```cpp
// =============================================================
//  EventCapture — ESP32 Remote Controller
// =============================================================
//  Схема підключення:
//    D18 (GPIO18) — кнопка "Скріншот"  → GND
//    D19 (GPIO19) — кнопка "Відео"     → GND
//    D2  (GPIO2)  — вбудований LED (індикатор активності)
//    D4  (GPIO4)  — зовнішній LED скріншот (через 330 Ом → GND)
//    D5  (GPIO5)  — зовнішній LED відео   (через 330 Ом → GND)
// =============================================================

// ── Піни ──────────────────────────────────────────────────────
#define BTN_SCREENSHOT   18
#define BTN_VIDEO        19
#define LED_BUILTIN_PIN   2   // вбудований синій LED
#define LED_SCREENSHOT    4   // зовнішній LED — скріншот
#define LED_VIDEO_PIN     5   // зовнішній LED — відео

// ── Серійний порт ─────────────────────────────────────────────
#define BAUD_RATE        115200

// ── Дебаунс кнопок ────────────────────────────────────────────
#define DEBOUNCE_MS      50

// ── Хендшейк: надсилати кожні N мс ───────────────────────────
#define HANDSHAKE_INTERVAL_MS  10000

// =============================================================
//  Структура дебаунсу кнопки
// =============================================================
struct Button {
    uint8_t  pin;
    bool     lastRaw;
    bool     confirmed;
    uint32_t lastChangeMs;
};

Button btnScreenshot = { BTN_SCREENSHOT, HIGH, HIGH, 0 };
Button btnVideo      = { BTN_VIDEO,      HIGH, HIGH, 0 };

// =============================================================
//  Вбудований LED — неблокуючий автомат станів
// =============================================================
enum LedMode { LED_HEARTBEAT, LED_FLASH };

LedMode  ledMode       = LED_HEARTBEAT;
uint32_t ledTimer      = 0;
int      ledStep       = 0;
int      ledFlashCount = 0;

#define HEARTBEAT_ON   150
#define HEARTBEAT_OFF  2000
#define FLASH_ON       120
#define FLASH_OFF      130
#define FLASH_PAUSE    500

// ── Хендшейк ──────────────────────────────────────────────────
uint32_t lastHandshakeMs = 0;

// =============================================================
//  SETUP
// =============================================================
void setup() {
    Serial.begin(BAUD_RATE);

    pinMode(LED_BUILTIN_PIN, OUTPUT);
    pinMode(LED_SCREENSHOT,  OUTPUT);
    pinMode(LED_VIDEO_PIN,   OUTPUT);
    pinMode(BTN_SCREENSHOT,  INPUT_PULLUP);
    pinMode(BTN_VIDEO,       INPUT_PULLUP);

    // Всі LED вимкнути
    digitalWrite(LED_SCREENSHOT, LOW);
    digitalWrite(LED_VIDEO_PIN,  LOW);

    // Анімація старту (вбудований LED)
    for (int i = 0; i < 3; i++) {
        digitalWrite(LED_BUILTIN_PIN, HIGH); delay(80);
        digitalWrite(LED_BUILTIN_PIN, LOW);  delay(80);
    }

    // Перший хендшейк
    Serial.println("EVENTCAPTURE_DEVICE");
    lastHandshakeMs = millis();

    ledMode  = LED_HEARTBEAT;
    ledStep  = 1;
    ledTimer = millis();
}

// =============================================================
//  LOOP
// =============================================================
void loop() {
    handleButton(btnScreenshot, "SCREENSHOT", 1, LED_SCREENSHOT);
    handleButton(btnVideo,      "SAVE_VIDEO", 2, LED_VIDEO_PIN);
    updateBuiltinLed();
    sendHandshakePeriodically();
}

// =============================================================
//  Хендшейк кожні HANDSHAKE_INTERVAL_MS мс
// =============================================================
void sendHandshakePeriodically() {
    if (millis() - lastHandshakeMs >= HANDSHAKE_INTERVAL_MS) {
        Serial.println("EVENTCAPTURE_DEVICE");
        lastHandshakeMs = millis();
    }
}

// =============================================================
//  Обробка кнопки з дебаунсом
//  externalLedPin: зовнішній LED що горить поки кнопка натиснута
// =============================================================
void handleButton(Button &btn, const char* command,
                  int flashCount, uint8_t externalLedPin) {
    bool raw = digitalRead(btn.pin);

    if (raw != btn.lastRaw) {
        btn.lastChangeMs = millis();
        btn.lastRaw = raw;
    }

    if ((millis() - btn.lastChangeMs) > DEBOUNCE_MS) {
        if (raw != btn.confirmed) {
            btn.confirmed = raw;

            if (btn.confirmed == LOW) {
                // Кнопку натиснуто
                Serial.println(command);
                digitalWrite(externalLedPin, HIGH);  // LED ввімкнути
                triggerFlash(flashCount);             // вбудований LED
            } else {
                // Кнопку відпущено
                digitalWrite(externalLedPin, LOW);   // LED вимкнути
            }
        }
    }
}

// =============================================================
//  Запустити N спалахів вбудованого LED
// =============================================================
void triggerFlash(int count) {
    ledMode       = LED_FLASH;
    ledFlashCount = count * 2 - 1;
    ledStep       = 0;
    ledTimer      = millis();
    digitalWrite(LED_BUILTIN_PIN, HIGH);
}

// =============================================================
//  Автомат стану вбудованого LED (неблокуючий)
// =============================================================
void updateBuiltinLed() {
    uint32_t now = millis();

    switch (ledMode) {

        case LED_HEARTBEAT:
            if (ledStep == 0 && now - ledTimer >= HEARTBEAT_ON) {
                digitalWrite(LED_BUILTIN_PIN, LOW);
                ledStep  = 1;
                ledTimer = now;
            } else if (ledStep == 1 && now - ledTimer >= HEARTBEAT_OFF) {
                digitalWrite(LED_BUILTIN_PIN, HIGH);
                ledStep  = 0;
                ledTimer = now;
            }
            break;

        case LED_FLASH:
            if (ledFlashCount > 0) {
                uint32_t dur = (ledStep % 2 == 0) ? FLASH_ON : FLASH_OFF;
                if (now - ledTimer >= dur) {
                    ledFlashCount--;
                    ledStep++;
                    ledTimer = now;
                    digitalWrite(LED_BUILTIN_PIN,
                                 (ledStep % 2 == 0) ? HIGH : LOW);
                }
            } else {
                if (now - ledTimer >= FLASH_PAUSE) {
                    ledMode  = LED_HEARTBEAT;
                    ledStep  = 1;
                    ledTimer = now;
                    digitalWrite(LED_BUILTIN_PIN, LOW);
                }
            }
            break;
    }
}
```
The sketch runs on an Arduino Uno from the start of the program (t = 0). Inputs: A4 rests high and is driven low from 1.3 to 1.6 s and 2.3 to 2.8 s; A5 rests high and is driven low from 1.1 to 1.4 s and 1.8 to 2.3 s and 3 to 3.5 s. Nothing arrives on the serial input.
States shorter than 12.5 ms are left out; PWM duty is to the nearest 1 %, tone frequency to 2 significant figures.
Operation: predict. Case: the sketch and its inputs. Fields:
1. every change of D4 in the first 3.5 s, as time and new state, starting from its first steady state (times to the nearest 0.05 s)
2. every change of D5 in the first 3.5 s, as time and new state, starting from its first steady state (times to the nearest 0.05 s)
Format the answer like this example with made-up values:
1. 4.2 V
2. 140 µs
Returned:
1. 0 s low; 1.35 s high; 1.65 s low; 2.35 s high; 2.85 s low
2. 0 s low; 1.15 s high; 1.45 s low; 1.85 s high; 2.35 s low; 3.05 s high
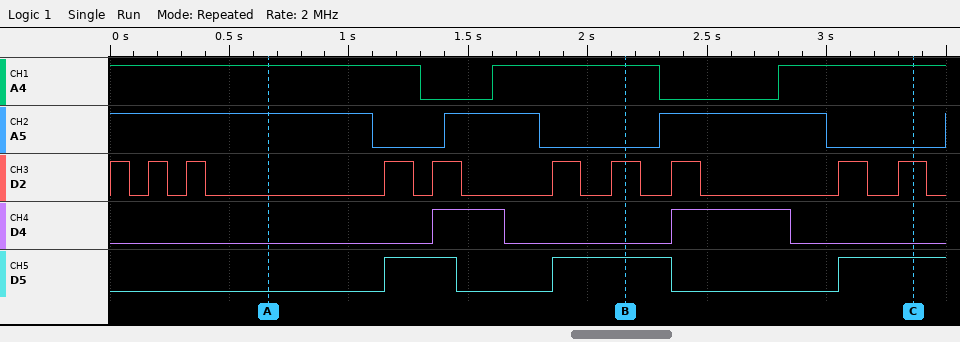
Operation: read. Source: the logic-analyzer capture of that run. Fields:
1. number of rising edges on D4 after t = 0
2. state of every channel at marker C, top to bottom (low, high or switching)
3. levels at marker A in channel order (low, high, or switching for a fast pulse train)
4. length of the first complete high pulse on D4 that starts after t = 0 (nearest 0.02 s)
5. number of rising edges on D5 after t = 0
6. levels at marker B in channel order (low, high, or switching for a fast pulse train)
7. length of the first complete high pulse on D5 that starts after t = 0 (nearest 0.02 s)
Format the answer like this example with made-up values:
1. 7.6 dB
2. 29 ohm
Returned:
1. 2
2. A4 high, A5 low, D2 high, D4 low, D5 high
3. A4 high, A5 high, D2 low, D4 low, D5 low
4. 0.30 s
5. 3
6. A4 high, A5 low, D2 high, D4 low, D5 high
7. 0.30 s
